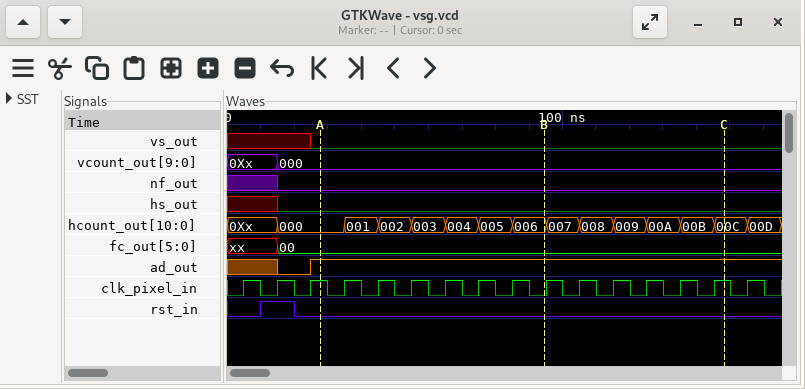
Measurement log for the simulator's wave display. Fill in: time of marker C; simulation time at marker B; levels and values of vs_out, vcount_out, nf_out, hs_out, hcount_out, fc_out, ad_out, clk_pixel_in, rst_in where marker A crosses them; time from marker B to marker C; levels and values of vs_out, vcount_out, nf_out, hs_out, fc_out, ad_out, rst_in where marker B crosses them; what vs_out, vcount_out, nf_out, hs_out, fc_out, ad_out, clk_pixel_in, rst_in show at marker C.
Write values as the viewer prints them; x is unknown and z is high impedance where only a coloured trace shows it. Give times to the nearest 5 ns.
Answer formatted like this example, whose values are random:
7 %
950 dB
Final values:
150 ns
95 ns
vs_out=0, vcount_out=000, nf_out=0, hs_out=0, hcount_out=000, fc_out=00, ad_out=1, clk_pixel_in=1, rst_in=0
55 ns
vs_out=0, vcount_out=000, nf_out=0, hs_out=0, fc_out=00, ad_out=1, rst_in=0
vs_out=0, vcount_out=000, nf_out=0, hs_out=0, fc_out=00, ad_out=1, clk_pixel_in=1, rst_in=0
